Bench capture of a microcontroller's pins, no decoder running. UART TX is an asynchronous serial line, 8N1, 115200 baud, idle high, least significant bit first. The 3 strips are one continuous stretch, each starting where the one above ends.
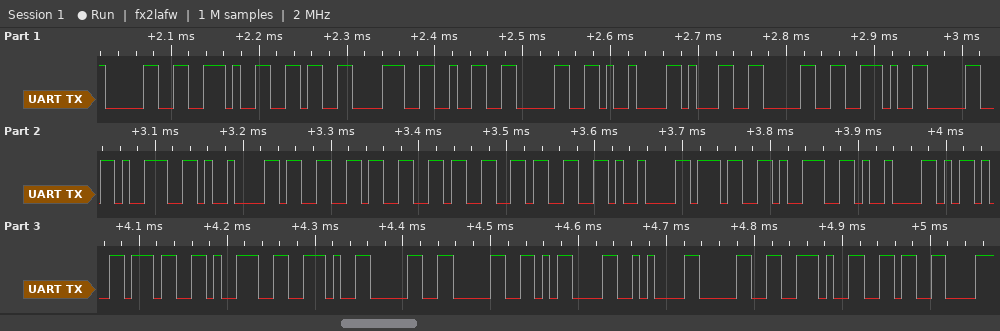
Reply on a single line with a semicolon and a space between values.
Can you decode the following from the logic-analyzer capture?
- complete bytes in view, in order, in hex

30 2E 36 38 32 30 09 31 30 2E 30 39 09 33 33 33 33 09 37 39 09 2D 37 39 2E 30 30 0D 0A 30 2E 36
